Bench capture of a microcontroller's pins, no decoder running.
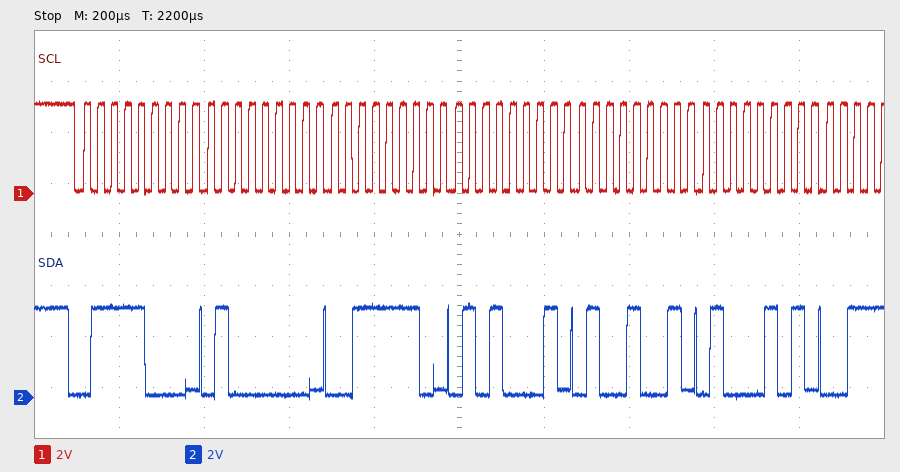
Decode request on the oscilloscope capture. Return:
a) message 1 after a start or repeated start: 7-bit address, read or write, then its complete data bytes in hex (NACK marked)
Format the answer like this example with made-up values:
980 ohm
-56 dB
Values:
0x3C write: 40 3E 51 49 45
